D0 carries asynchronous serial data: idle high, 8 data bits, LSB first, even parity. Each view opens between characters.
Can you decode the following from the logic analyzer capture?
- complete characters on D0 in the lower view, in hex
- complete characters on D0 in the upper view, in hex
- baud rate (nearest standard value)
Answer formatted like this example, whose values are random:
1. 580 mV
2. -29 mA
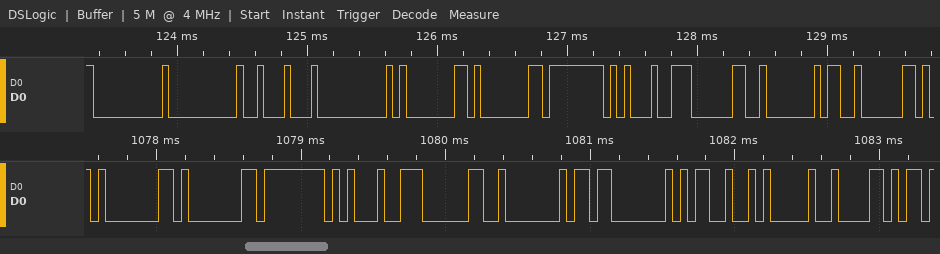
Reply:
1. 01, 01, FF, 91, 60, 40, 03, 4D, 41, 58
2. 00, 00, 22, 00, 01, 01, FF, 91, 60, 40, 02
3. 19200 baud
